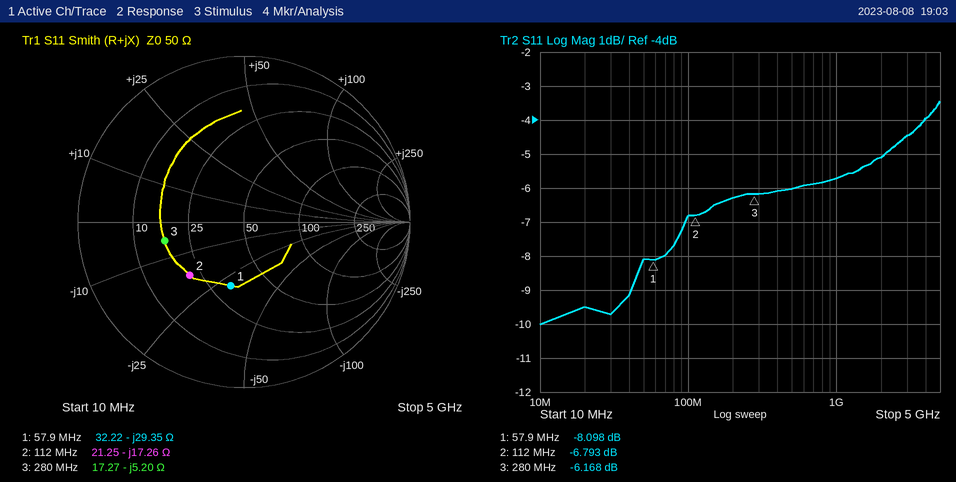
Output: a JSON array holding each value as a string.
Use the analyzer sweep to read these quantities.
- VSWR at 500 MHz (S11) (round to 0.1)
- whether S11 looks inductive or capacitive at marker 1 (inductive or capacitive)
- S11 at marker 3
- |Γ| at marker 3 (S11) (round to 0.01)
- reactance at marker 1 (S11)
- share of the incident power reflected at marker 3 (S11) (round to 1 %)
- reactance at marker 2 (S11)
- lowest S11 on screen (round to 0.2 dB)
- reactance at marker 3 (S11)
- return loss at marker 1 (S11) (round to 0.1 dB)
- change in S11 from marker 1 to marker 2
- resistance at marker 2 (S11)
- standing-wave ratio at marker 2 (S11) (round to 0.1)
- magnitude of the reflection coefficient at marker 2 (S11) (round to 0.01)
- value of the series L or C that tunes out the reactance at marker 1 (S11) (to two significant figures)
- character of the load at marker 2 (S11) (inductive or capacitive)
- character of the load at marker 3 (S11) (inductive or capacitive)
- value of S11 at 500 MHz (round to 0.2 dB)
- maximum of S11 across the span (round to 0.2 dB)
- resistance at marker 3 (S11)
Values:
["3.0", "capacitive", "-6.168 dB", "0.49", "-29.35 Ω", "24 %", "-17.26 Ω", "-10.0 dB", "-5.20 Ω", "8.1 dB", "1.305 dB", "21.25 Ω", "2.7", "0.46", "81 nH", "capacitive", "capacitive", "-6.0 dB", "-3.4 dB", "17.27 Ω"]
